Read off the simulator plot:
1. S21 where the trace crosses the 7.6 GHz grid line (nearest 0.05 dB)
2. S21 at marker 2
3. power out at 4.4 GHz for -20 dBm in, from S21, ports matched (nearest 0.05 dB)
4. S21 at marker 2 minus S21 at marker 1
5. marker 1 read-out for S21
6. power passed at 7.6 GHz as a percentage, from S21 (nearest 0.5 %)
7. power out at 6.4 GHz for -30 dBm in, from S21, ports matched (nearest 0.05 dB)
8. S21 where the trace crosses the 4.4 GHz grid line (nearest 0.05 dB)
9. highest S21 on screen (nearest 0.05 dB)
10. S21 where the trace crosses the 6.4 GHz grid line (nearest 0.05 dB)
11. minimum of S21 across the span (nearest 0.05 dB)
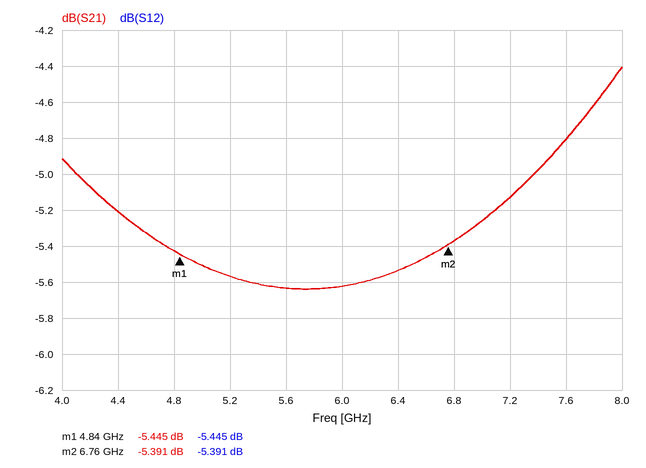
-4.80 dB
-5.391 dB
-25.20 dBm
0.054 dB
-5.445 dB
33.0 %
-35.55 dBm
-5.20 dB
-4.40 dB
-5.55 dB
-5.65 dB
